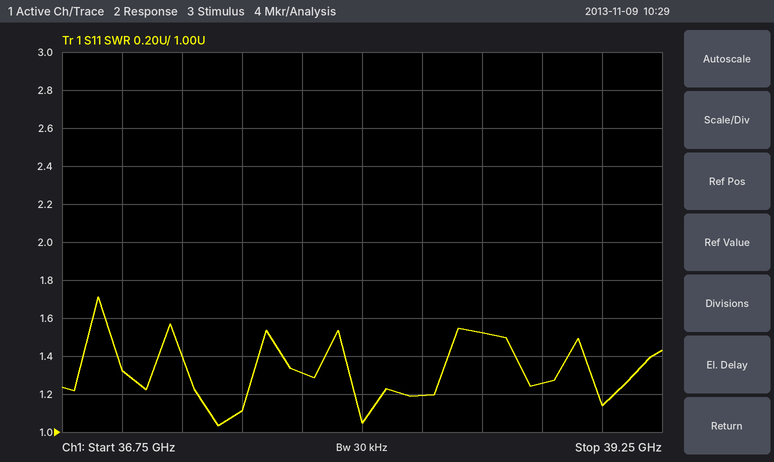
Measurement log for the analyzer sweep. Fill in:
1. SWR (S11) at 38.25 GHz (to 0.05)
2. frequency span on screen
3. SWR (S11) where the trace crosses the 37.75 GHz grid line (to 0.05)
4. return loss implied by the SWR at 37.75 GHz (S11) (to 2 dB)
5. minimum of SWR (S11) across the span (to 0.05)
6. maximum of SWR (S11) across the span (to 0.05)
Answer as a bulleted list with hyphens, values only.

- 1.20
- 2.5 GHz
- 1.30
- 18 dB
- 1.05
- 1.70
